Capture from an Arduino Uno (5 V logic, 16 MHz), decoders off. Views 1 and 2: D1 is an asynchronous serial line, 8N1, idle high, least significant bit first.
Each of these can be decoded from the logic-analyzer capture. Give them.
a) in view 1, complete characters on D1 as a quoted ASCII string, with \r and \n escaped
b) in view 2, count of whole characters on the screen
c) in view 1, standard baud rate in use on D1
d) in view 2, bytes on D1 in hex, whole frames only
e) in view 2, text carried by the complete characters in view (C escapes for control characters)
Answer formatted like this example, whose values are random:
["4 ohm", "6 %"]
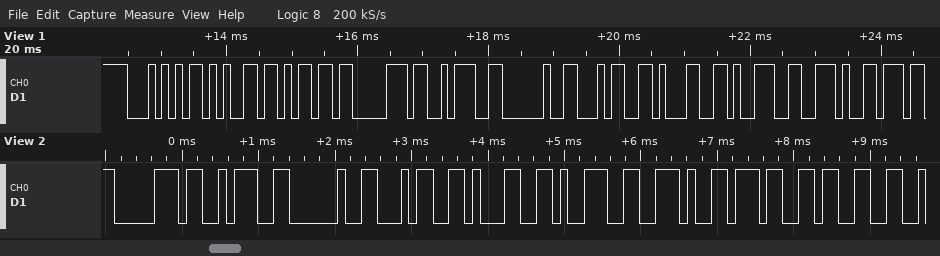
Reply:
["\"Temp: 419.\"", "9", "9600 baud", "0x70 0x3A 0x20 0x34 0x31 0x39 0x2E 0x37 0x33", "\"p: 419.73\""]
